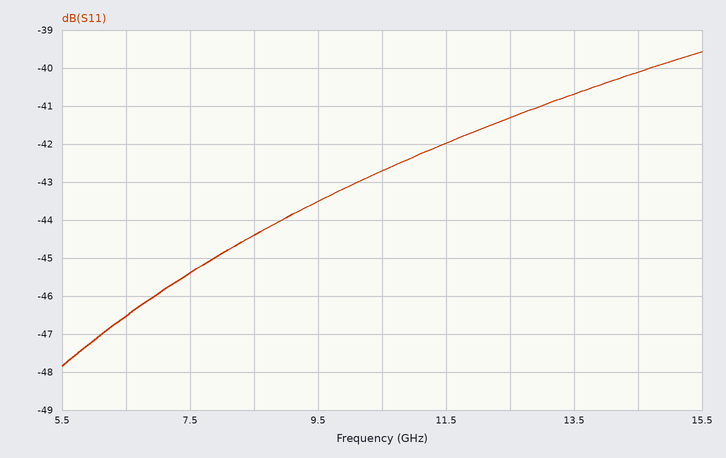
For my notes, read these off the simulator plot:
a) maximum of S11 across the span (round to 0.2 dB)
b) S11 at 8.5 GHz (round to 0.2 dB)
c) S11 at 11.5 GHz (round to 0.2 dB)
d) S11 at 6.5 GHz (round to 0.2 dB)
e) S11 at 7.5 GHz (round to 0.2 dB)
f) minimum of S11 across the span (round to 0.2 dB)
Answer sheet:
-39.6 dB
-44.4 dB
-42.0 dB
-46.6 dB
-45.4 dB
-47.8 dB
